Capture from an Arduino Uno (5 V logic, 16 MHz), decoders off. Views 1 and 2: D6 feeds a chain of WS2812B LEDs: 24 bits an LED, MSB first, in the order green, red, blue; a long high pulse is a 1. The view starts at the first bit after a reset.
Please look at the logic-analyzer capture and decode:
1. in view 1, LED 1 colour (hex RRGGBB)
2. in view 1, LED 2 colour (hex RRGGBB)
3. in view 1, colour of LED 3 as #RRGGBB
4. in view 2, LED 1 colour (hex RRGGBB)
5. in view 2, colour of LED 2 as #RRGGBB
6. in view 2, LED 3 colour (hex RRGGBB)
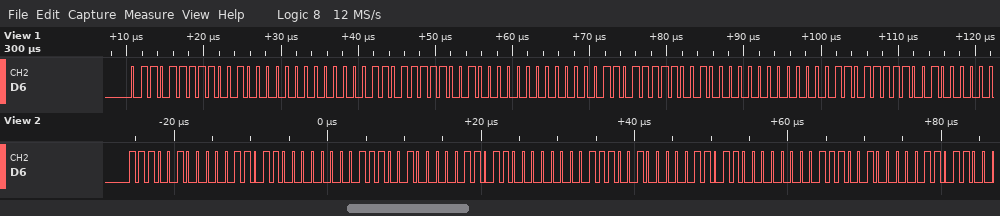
#906F00
#906F00
#906F00
#1BE400
#1BE400
#1BE400
